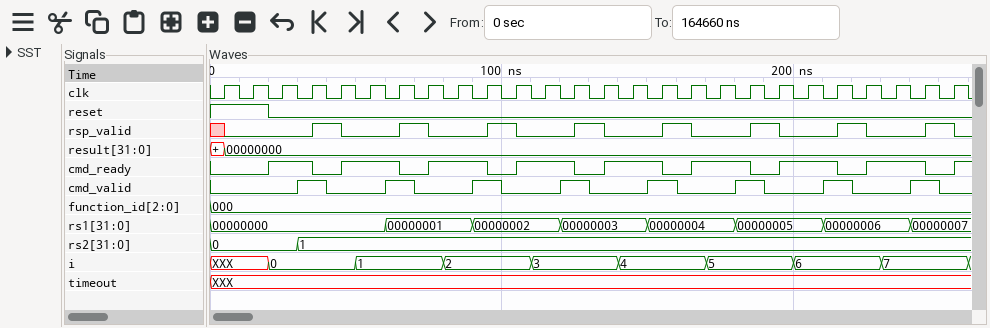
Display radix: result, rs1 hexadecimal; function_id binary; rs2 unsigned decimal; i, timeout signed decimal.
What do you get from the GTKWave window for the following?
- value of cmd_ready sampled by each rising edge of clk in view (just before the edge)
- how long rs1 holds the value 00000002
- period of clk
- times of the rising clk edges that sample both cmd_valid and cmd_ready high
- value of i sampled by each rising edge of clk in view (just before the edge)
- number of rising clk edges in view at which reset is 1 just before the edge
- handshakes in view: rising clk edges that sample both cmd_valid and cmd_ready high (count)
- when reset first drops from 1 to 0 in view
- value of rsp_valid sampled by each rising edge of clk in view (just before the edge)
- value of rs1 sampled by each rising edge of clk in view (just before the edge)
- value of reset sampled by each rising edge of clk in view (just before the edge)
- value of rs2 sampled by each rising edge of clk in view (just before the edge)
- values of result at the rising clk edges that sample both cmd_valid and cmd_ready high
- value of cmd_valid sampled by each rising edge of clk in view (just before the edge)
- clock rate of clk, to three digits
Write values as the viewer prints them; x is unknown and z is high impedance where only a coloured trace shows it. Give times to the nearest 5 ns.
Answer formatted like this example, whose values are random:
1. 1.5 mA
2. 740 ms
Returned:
1. 0 0 1 1 0 1 1 0 1 1 0 1 1 0 1 1 0 1 1 0 1 1 0 1 1 0
2. 30 ns
3. 10 ns
4. 35 ns, 65 ns, 95 ns, 125 ns, 155 ns, 185 ns, 215 ns, 245 ns
5. XXX, XXX, 0, 0, 0, 1, 1, 1, 2, 2, 2, 3, 3, 3, 4, 4, 4, 5, 5, 5, 6, 6, 6, 7, 7, 7
6. 2
7. 8
8. 20 ns
9. x 0 0 0 1 0 0 1 0 0 1 0 0 1 0 0 1 0 0 1 0 0 1 0 0 1
10. 00000000, 00000000, 00000000, 00000000, 00000000, 00000000, 00000001, 00000001, 00000001, 00000002, 00000002, 00000002, 00000003, 00000003, 00000003, 00000004, 00000004, 00000004, 00000005, 00000005, 00000005, 00000006, 00000006, 00000006, 00000007, 00000007
11. 1 1 0 0 0 0 0 0 0 0 0 0 0 0 0 0 0 0 0 0 0 0 0 0 0 0
12. 0, 0, 0, 1, 1, 1, 1, 1, 1, 1, 1, 1, 1, 1, 1, 1, 1, 1, 1, 1, 1, 1, 1, 1, 1, 1
13. 00000000, 00000000, 00000000, 00000000, 00000000, 00000000, 00000000, 00000000
14. 0 0 0 1 0 0 1 0 0 1 0 0 1 0 0 1 0 0 1 0 0 1 0 0 1 0
15. 100 MHz
